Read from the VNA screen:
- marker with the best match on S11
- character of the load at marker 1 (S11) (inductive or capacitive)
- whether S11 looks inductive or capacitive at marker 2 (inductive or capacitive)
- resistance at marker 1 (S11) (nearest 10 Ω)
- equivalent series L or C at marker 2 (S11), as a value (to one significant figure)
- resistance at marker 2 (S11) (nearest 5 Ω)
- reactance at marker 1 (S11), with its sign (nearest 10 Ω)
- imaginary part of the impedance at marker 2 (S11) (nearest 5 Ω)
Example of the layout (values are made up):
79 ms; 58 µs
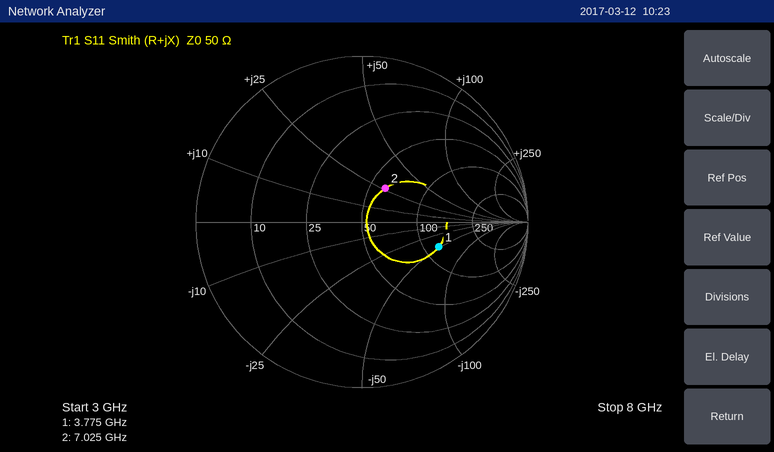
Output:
marker 2; capacitive; inductive; 120 Ω; 600 pH; 60 Ω; -50 Ω; +25 Ω
